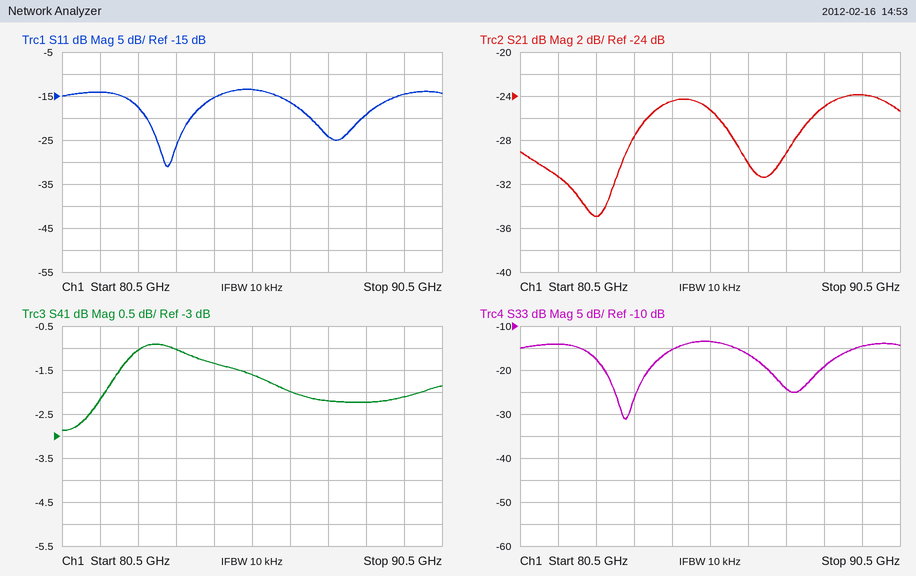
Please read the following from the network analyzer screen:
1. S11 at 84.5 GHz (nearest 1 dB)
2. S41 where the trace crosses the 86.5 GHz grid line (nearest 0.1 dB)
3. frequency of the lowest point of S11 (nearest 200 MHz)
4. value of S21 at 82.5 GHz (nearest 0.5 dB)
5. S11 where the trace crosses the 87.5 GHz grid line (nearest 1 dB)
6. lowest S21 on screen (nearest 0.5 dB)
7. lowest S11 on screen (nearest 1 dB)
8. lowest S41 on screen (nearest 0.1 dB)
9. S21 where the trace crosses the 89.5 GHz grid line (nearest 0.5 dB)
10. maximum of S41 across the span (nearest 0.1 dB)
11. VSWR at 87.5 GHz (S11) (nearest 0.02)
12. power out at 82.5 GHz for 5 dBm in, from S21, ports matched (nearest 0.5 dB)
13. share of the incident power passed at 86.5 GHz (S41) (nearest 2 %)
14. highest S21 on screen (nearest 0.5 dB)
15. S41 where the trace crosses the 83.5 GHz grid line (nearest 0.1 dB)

-15 dB
-2.0 dB
83.2 GHz
-35.0 dB
-24 dB
-35.0 dB
-31 dB
-2.9 dB
-24.0 dB
-0.9 dB
1.14
-30.0 dBm
64 %
-24.0 dB
-1.0 dB
